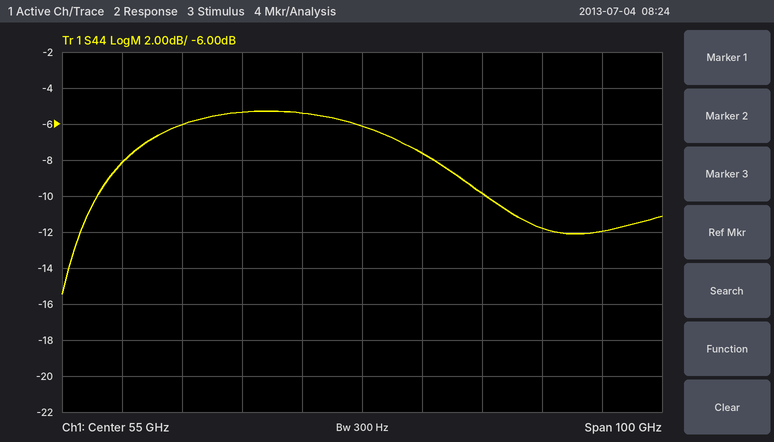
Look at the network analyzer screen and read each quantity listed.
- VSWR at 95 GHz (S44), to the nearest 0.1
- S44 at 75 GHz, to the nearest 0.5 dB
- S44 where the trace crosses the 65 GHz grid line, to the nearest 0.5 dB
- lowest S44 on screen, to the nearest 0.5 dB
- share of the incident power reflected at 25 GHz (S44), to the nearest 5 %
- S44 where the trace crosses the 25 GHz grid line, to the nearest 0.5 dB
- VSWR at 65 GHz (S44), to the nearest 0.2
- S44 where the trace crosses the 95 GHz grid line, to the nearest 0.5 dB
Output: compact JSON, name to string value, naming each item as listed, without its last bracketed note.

{"VSWR at 95 GHz (S44), to the nearest 0.1": "1.7", "S44 at 75 GHz, to the nearest 0.5 dB": "-10.0 dB", "S44 where the trace crosses the 65 GHz grid line, to the nearest 0.5 dB": "-7.5 dB", "lowest S44 on screen, to the nearest 0.5 dB": "-15.5 dB", "share of the incident power reflected at 25 GHz (S44), to the nearest 5 %": "25 %", "S44 where the trace crosses the 25 GHz grid line, to the nearest 0.5 dB": "-6.0 dB", "VSWR at 65 GHz (S44), to the nearest 0.2": "2.4", "S44 where the trace crosses the 95 GHz grid line, to the nearest 0.5 dB": "-12.0 dB"}
